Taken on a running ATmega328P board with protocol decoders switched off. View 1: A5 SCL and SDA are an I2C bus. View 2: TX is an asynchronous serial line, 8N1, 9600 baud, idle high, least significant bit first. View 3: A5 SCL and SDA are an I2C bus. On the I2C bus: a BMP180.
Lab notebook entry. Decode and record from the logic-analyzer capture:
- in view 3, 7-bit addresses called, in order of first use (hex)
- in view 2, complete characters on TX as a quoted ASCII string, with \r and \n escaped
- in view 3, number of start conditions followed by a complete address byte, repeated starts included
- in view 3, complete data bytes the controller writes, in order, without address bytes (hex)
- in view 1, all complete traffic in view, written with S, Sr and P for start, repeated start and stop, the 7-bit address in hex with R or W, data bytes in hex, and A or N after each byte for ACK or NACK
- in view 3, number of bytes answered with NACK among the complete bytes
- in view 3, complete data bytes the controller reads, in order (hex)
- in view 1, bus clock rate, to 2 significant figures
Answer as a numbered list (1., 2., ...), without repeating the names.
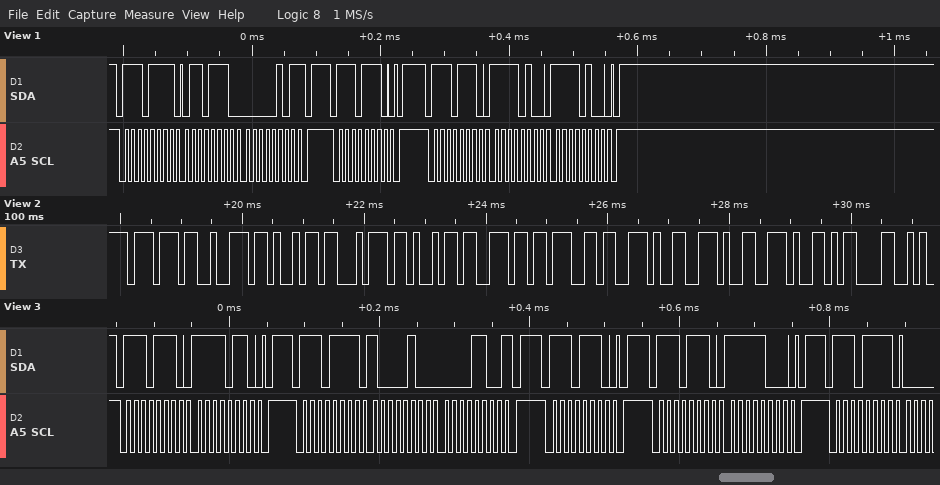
1. 0x77
2. "writing...\r"
3. 5
4. F6 F8
5. S 77R A 6E A 05 N P S 77W A P S 77W A F4 A F4 A P
6. 1
7. 84 0C
8. 100 kHz
